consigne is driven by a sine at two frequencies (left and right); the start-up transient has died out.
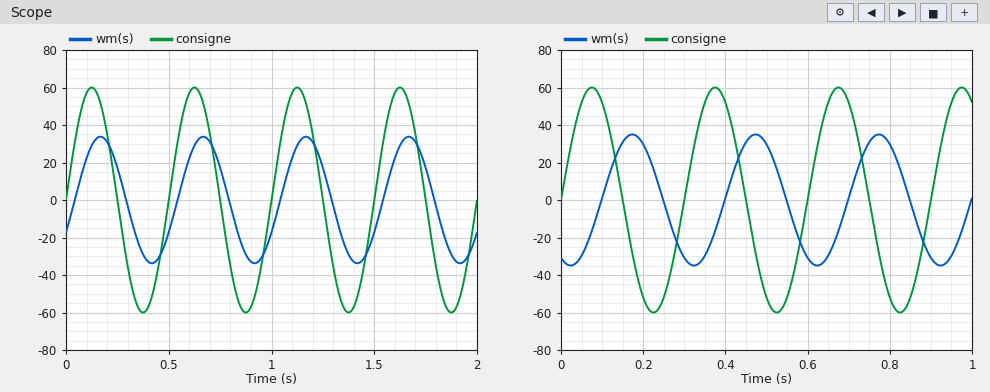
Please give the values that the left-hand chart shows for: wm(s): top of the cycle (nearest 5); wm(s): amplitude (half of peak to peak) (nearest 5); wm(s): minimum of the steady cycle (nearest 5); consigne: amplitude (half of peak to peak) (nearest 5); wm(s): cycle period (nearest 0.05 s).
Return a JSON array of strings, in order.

["35", "35", "-35", "60", "0.50 s"]
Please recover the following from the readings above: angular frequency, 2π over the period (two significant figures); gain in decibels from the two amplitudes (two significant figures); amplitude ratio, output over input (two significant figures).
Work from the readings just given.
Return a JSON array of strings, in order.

["13 rad/s", "-4.7 dB", "0.58"]
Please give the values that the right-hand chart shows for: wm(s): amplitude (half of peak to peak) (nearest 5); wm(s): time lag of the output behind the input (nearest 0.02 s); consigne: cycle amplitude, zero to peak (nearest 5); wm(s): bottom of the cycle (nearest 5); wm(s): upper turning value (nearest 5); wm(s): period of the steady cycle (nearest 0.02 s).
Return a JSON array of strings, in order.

["35", "0.10 s", "60", "-35", "35", "0.30 s"]
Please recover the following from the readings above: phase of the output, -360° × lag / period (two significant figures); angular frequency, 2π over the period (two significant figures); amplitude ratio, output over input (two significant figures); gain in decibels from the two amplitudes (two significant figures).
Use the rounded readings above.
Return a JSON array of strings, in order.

["-120°", "21 rad/s", "0.58", "-4.7 dB"]
